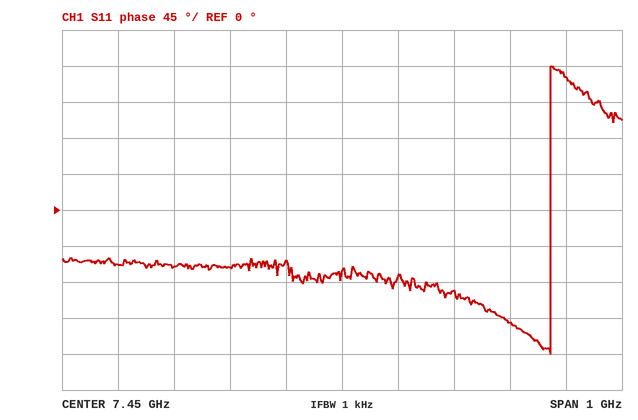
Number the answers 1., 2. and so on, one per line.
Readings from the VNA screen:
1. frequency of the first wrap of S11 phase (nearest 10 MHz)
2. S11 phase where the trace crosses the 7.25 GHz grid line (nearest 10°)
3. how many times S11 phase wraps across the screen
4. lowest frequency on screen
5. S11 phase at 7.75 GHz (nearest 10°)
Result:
1. 7.82 GHz
2. -70°
3. 1
4. 6.95 GHz
5. -140°
